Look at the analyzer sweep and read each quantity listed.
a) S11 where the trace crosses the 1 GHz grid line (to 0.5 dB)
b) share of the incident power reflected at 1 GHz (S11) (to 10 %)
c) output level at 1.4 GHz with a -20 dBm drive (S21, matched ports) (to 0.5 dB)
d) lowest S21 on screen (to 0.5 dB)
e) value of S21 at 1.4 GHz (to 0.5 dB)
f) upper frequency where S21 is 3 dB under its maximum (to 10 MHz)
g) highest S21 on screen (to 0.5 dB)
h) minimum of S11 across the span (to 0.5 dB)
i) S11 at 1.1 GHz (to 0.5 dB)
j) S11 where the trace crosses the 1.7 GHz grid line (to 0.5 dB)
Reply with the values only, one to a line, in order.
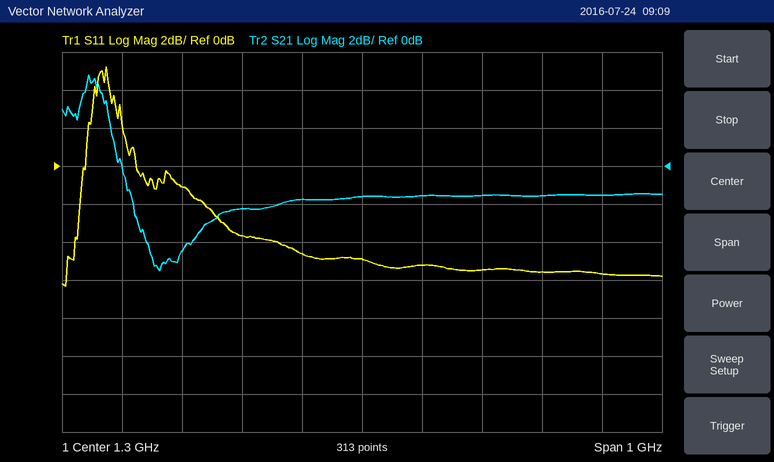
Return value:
-1.0 dB
80 %
-21.5 dBm
-5.5 dB
-1.5 dB
880 MHz
5.0 dB
-6.5 dB
-3.5 dB
-5.5 dB
